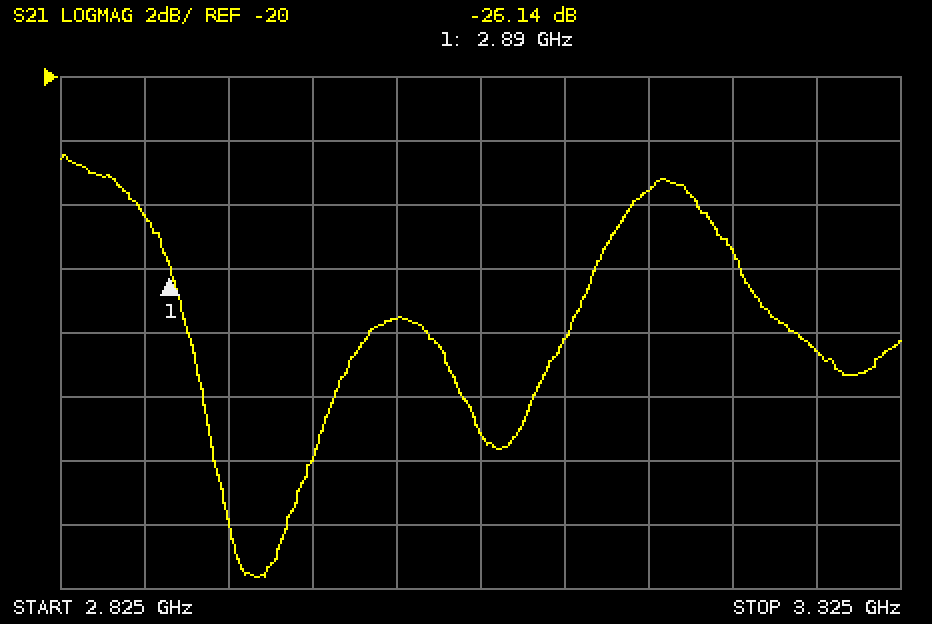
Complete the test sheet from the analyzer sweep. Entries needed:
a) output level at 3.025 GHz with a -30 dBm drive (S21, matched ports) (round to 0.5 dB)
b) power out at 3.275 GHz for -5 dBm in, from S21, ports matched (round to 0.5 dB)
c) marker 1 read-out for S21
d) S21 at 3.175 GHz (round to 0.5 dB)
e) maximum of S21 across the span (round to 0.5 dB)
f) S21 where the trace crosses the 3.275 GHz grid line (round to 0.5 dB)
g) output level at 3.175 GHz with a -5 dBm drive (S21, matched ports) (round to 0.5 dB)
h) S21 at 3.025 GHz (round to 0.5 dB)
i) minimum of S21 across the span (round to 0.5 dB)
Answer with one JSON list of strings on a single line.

["-57.5 dBm", "-33.5 dBm", "-26.14 dB", "-23.5 dB", "-22.5 dB", "-28.5 dB", "-28.5 dBm", "-27.5 dB", "-35.5 dB"]
